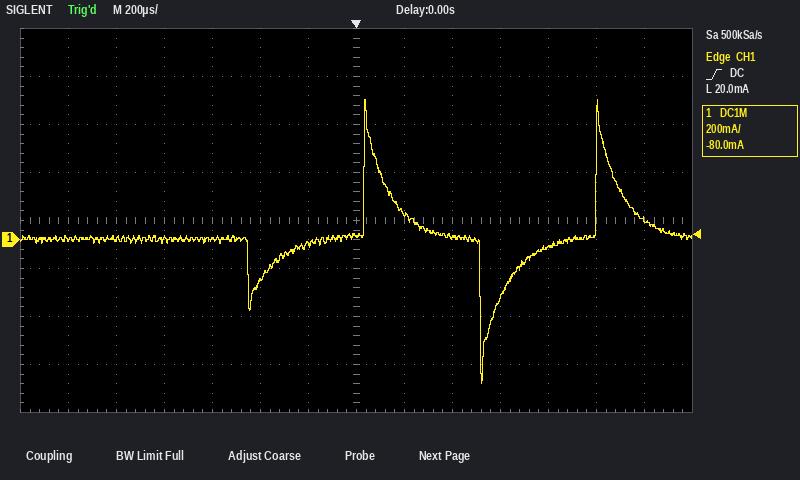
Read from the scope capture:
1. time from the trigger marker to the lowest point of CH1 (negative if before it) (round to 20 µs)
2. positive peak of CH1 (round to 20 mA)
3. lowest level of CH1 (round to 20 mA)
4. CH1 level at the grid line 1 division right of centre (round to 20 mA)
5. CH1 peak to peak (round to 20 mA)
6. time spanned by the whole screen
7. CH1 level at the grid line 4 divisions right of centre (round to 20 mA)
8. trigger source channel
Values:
+520 µs
580 mA
-600 mA
100 mA
1.18 A
2.8 ms
-40 mA
CH1
